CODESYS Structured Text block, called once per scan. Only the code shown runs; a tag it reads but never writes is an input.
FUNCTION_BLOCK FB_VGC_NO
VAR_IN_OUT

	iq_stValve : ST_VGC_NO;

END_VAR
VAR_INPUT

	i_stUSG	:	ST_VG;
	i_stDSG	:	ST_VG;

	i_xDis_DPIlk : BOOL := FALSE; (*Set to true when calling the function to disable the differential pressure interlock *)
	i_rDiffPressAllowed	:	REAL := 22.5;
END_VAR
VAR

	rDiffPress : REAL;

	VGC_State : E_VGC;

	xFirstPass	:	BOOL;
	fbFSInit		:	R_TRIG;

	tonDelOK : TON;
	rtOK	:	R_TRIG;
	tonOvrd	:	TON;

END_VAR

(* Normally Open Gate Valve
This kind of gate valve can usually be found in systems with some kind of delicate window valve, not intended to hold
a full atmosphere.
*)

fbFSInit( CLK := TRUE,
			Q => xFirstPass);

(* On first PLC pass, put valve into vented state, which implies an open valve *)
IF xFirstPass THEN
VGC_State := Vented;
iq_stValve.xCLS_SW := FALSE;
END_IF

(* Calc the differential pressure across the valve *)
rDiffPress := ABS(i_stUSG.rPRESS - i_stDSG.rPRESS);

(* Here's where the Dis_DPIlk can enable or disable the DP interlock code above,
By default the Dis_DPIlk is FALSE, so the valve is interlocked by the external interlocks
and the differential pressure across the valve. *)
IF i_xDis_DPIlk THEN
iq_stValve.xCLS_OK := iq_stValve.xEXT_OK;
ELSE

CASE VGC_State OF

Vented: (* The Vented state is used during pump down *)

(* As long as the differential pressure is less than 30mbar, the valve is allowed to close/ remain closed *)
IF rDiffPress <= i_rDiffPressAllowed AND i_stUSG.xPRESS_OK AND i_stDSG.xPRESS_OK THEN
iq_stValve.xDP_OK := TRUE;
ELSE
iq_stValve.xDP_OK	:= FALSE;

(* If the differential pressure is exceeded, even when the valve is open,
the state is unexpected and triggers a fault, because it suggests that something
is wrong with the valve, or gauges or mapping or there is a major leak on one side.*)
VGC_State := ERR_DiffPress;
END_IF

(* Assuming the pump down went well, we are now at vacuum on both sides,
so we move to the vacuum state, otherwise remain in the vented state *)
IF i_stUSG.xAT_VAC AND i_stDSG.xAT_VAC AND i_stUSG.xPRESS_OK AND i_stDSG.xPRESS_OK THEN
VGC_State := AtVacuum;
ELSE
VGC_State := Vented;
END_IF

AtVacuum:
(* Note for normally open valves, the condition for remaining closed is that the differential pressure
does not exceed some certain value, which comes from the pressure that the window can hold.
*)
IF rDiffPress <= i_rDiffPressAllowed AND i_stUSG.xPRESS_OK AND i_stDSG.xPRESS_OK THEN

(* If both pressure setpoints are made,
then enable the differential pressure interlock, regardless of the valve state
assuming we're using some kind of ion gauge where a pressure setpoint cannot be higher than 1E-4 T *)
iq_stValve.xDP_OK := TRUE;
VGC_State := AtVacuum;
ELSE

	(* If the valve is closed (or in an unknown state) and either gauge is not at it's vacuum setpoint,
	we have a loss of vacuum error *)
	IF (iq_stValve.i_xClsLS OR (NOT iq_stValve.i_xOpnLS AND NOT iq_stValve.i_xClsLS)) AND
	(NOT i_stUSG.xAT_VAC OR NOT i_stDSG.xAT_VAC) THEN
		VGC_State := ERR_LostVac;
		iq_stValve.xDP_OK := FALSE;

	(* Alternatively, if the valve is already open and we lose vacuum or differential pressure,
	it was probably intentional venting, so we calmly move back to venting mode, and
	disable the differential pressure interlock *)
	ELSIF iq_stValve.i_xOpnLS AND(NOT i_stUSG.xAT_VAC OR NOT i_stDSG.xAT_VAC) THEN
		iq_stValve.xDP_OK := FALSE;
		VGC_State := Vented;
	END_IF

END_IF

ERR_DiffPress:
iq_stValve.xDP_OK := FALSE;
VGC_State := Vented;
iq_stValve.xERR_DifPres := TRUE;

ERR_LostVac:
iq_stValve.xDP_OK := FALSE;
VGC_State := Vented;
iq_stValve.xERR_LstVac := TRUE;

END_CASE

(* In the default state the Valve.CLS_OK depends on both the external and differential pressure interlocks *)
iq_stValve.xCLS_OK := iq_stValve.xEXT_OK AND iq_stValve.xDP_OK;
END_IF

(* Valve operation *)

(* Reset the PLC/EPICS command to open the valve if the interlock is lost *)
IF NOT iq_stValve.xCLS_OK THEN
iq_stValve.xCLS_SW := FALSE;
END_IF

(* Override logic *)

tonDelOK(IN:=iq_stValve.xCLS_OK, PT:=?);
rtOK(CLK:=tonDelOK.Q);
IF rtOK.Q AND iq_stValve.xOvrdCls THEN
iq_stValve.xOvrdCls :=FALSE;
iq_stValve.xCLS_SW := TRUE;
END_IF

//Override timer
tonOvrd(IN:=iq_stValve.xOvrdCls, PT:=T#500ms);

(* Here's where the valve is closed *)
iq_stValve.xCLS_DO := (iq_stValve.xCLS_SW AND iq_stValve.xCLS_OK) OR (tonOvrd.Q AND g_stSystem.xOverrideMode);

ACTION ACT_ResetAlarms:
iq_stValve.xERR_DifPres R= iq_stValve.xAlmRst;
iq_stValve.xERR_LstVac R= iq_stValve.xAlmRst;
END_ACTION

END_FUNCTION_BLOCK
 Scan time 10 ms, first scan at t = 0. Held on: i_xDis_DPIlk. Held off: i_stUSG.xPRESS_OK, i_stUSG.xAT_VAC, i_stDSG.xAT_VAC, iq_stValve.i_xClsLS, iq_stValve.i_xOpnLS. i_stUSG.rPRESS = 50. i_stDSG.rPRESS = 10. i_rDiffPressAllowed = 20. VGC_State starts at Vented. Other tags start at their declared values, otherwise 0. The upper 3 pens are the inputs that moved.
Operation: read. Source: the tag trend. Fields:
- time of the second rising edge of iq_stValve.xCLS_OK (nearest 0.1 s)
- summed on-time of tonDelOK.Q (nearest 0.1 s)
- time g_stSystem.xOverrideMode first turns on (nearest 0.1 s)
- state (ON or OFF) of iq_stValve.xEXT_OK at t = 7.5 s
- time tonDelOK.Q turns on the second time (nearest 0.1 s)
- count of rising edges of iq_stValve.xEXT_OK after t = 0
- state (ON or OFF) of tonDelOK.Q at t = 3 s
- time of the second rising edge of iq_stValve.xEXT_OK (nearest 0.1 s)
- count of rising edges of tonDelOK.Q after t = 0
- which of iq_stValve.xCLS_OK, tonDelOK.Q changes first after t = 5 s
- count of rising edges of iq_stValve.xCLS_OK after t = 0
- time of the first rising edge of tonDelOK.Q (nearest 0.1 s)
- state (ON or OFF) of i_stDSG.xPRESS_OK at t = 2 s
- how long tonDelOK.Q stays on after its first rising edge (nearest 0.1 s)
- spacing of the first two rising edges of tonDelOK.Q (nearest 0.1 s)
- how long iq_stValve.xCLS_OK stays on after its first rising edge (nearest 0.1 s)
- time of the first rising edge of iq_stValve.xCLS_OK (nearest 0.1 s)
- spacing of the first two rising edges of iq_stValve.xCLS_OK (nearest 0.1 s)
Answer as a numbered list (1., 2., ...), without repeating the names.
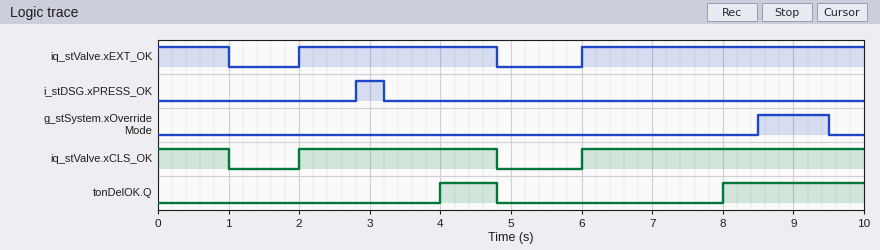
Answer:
1. 6.0 s
2. 2.8 s
3. 8.5 s
4. ON
5. 8.0 s
6. 2
7. OFF
8. 6.0 s
9. 2
10. iq_stValve.xCLS_OK
11. 2
12. 4.0 s
13. OFF
14. 0.8 s
15. 4.0 s
16. 2.8 s
17. 2.0 s
18. 4.0 s
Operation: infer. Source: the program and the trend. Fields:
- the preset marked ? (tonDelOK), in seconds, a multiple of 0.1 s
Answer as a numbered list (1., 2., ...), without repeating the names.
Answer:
1. 2.0 s
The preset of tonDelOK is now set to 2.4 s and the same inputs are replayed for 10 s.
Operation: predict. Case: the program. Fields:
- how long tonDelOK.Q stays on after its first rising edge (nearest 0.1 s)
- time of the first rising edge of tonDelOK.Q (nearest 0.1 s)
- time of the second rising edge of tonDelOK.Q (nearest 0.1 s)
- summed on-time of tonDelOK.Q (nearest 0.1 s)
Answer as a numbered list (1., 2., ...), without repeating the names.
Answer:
1. 0.4 s
2. 4.4 s
3. 8.4 s
4. 2.0 s
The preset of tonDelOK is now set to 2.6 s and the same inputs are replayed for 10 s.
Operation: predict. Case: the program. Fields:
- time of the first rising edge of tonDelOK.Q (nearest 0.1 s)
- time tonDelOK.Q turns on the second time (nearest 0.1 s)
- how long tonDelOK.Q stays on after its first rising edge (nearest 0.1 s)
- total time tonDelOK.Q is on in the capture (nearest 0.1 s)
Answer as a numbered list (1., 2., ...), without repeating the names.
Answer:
1. 4.6 s
2. 8.6 s
3. 0.2 s
4. 1.6 s
